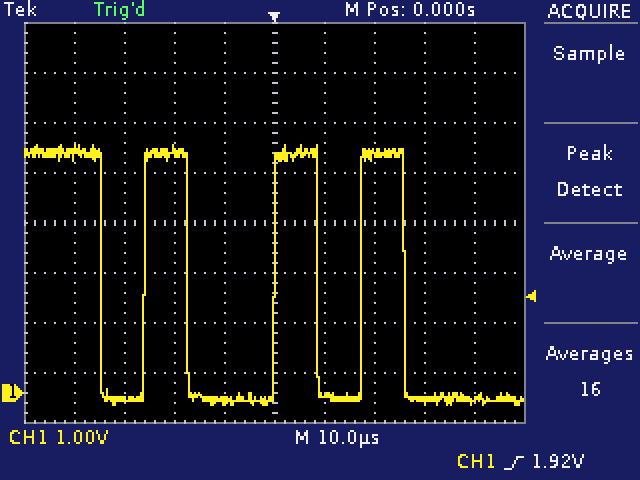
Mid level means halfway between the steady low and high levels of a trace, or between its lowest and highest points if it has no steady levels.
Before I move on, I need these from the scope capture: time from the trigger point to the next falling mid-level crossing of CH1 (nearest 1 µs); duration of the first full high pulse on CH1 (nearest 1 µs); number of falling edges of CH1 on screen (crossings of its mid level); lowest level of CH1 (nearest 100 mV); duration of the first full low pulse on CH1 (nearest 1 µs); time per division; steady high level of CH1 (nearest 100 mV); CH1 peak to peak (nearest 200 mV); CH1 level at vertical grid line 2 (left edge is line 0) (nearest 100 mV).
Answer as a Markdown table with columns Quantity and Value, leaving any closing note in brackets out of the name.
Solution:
| Quantity | Value |
|---|---|
| time from the trigger point to the next falling mid-level crossing of CH1 | 9 µs |
| duration of the first full high pulse on CH1 | 9 µs |
| number of falling edges of CH1 on screen | 4 |
| lowest level of CH1 | -200 mV |
| duration of the first full low pulse on CH1 | 9 µs |
| time per division | 10 µs |
| steady high level of CH1 | 4.8 V |
| CH1 peak to peak | 5.2 V |
| CH1 level at vertical grid line 2 (left edge is line 0) | -100 mV |
